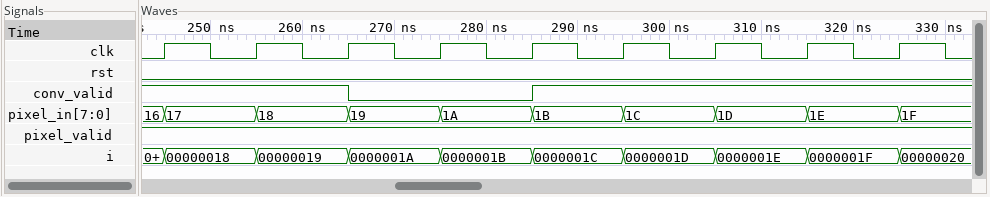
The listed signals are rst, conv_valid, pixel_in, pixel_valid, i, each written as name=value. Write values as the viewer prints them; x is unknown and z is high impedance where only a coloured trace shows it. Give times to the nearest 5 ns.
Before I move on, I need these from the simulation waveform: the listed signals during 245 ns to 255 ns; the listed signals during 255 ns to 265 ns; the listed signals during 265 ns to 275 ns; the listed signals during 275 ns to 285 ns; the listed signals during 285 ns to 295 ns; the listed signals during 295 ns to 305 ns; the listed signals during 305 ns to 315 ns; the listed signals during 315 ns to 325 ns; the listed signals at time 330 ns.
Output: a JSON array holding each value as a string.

["rst=0, conv_valid=1, pixel_in=17, pixel_valid=1, i=00000018", "rst=0, conv_valid=1, pixel_in=18, pixel_valid=1, i=00000019", "rst=0, conv_valid=0, pixel_in=19, pixel_valid=1, i=0000001A", "rst=0, conv_valid=0, pixel_in=1A, pixel_valid=1, i=0000001B", "rst=0, conv_valid=1, pixel_in=1B, pixel_valid=1, i=0000001C", "rst=0, conv_valid=1, pixel_in=1C, pixel_valid=1, i=0000001D", "rst=0, conv_valid=1, pixel_in=1D, pixel_valid=1, i=0000001E", "rst=0, conv_valid=1, pixel_in=1E, pixel_valid=1, i=0000001F", "rst=0, conv_valid=1, pixel_in=1F, pixel_valid=1, i=00000020"]
